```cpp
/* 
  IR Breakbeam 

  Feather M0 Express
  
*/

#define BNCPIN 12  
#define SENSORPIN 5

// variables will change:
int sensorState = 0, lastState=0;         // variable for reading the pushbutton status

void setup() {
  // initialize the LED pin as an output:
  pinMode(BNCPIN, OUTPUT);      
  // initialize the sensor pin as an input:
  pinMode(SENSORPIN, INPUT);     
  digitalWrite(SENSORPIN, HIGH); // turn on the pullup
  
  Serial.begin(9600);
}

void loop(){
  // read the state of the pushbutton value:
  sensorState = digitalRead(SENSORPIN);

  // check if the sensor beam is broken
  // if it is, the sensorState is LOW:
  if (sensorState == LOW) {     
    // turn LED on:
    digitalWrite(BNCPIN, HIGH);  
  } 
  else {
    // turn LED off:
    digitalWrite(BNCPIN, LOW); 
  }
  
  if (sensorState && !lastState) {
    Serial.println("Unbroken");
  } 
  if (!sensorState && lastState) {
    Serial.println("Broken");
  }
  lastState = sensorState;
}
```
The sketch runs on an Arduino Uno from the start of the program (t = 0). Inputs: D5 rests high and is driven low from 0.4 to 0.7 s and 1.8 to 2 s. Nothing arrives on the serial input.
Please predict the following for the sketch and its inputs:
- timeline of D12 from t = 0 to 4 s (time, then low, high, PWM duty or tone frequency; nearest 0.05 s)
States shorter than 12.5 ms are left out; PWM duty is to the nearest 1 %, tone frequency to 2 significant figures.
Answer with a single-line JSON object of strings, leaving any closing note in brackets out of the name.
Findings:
{"timeline of D12 from t = 0 to 4 s": "0 s low; 0.4 s high; 0.7 s low; 1.8 s high; 2 s low"}
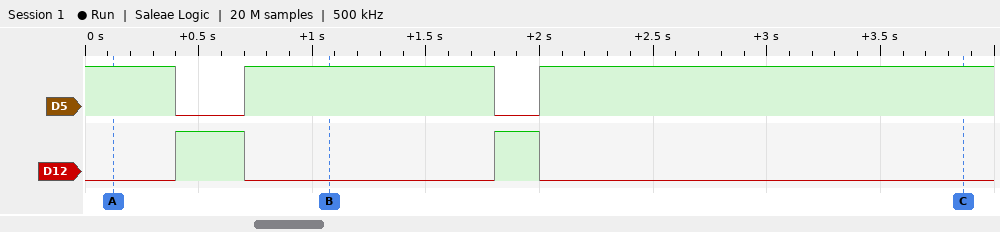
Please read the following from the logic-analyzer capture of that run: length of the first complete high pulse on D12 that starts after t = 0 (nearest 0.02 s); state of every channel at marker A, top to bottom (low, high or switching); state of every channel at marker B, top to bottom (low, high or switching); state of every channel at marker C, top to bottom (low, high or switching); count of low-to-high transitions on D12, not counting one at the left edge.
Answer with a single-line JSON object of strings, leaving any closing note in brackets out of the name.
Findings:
{"length of the first complete high pulse on D12 that starts after t = 0": "0.30 s", "state of every channel at marker A, top to bottom": "D5 high, D12 low", "state of every channel at marker B, top to bottom": "D5 high, D12 low", "state of every channel at marker C, top to bottom": "D5 high, D12 low", "count of low-to-high transitions on D12, not counting one at the left edge": "2"}
